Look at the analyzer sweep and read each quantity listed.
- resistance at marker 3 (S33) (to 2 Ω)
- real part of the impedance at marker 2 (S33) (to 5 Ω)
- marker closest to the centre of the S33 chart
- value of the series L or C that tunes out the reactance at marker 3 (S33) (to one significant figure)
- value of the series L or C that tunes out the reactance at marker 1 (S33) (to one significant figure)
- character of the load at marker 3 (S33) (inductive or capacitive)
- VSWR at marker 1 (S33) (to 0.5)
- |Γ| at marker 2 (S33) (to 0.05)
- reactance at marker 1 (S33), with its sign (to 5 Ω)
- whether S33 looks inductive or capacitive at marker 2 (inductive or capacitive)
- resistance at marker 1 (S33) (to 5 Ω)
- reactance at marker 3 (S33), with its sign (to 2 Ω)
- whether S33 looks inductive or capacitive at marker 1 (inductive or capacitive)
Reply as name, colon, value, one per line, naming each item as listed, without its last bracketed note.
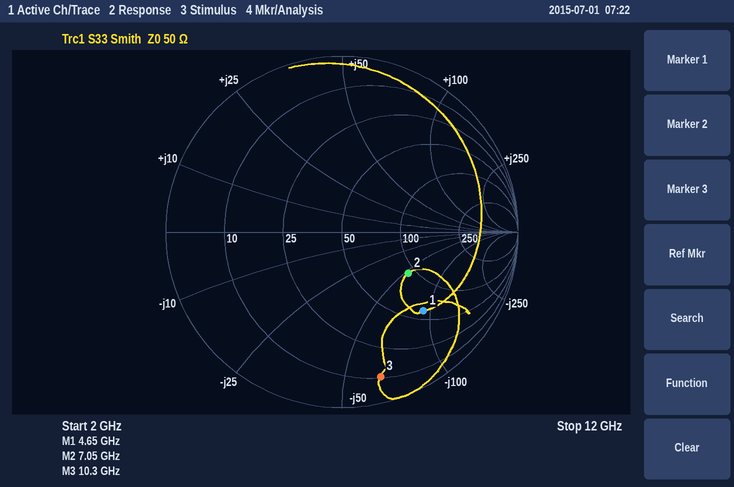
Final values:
resistance at marker 3 (S33): 10 Ω
real part of the impedance at marker 2 (S33): 90 Ω
marker closest to the centre of the S33 chart: marker 2
value of the series L or C that tunes out the reactance at marker 3 (S33): 1.0 nH
value of the series L or C that tunes out the reactance at marker 1 (S33): 3 nH
character of the load at marker 3 (S33): capacitive
VSWR at marker 1 (S33): 4.5
|Γ| at marker 2 (S33): 0.45
reactance at marker 1 (S33), with its sign: -90 Ω
whether S33 looks inductive or capacitive at marker 2: capacitive
resistance at marker 1 (S33): 60 Ω
reactance at marker 3 (S33), with its sign: -64 Ω
whether S33 looks inductive or capacitive at marker 1: capacitive
